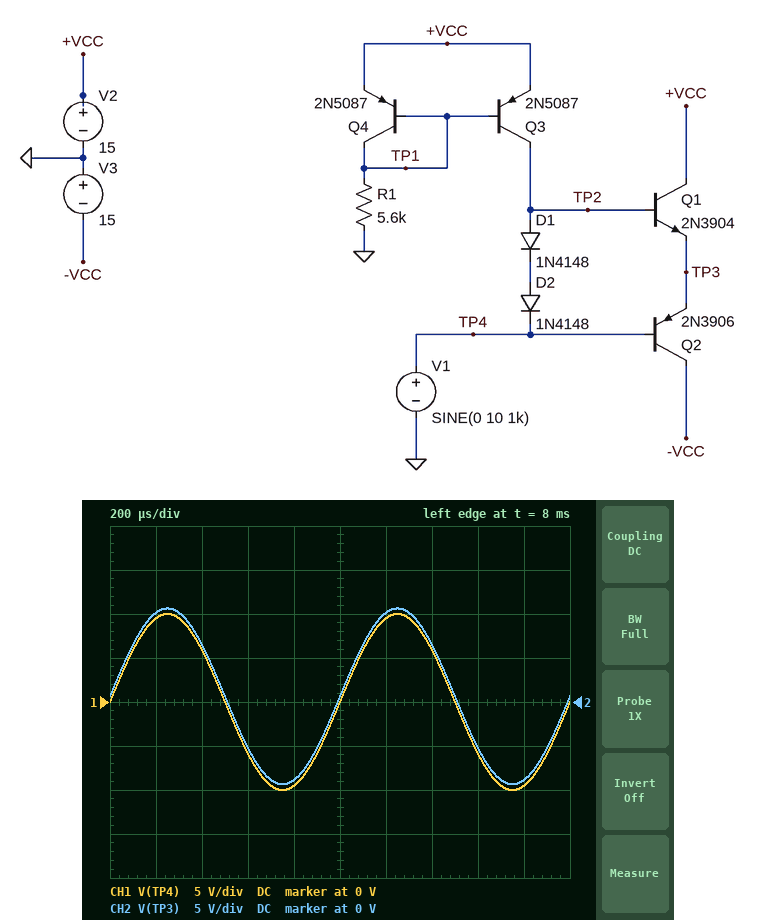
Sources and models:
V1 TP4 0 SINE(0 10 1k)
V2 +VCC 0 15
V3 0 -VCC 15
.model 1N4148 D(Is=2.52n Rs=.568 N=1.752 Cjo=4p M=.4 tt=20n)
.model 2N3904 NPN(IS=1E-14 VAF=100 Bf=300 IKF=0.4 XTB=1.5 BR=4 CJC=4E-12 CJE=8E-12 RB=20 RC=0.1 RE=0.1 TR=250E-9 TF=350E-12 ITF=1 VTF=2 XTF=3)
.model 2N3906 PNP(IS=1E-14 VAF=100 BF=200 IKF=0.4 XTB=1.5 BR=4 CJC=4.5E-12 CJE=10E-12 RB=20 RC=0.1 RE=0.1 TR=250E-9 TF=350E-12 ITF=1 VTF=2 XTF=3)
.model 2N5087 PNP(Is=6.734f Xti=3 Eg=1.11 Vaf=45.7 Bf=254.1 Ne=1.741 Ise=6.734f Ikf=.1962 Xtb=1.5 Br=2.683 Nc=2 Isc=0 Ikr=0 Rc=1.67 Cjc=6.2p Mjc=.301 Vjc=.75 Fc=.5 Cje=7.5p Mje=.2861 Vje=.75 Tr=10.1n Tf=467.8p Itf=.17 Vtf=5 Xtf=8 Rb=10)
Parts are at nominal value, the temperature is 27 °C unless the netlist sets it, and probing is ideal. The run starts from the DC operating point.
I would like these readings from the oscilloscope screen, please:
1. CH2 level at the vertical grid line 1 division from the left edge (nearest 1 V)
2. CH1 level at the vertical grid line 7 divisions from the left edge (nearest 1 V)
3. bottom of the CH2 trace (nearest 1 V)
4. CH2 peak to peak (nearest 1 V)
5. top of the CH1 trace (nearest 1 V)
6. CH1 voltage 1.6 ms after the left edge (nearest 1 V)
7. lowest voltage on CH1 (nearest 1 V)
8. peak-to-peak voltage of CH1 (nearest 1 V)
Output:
10 V
6 V
-9 V
20 V
10 V
-6 V
-10 V
20 V
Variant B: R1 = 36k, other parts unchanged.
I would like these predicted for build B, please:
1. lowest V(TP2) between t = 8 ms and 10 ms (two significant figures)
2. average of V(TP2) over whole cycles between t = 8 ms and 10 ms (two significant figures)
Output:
-8.9 V
1.1 V
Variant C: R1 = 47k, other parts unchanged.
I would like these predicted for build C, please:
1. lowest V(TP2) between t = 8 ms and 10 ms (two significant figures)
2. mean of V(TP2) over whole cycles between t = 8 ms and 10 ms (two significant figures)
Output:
-8.9 V
1.1 V
